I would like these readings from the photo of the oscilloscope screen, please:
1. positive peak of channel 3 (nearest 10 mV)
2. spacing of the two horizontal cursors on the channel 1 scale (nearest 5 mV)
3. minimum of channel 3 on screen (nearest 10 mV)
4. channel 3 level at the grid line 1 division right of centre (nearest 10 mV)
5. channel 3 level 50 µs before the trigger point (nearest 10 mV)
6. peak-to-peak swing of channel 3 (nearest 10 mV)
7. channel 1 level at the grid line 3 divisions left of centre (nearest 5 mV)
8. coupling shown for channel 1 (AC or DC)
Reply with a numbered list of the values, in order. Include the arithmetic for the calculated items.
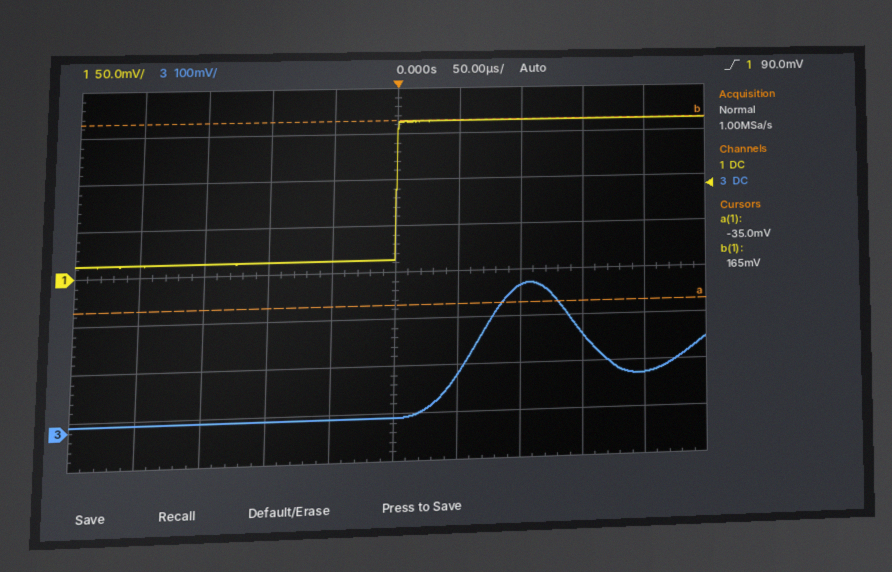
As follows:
1. 290 mV
2. 200 mV
3. 10 mV
4. 100 mV
5. 10 mV
6. 290 mV − (10 mV) = 280 mV
7. 15 mV
8. DC
